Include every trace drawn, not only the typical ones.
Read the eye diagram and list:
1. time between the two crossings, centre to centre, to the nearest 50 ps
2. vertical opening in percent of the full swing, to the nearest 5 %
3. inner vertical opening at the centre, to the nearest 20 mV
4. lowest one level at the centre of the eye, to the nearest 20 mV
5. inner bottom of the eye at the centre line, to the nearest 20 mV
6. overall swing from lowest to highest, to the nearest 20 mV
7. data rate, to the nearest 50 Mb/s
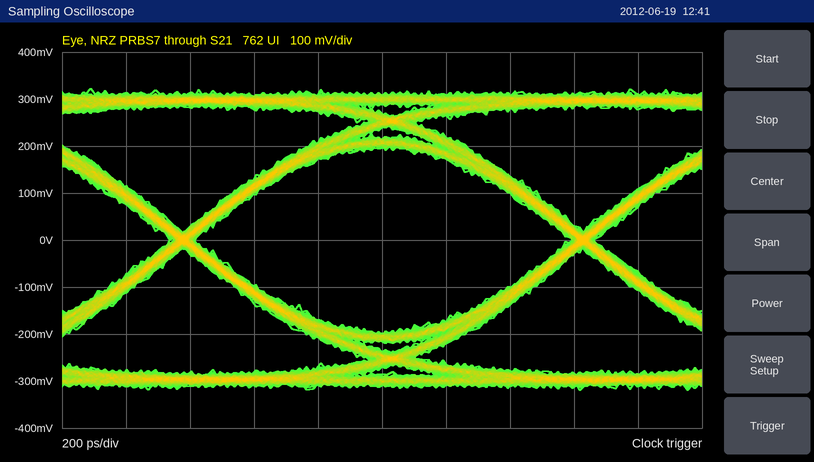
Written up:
1.25 ns
60 %
400 mV
200 mV
-200 mV
640 mV
800 Mb/s
